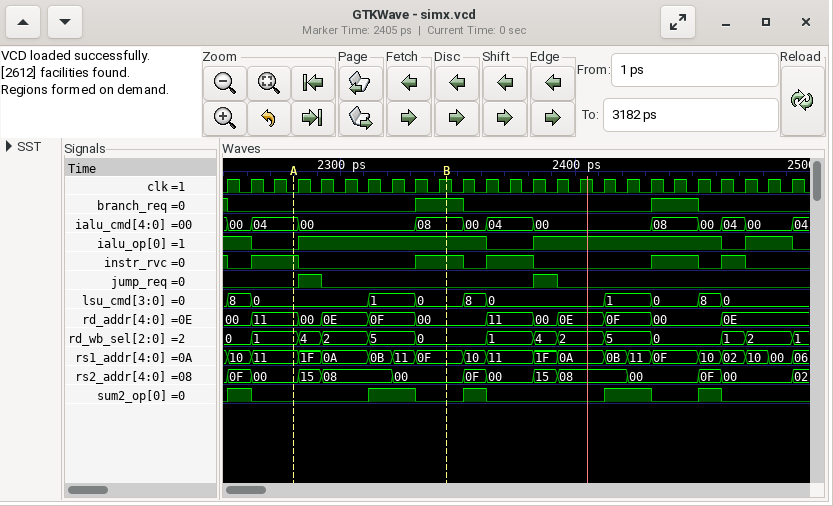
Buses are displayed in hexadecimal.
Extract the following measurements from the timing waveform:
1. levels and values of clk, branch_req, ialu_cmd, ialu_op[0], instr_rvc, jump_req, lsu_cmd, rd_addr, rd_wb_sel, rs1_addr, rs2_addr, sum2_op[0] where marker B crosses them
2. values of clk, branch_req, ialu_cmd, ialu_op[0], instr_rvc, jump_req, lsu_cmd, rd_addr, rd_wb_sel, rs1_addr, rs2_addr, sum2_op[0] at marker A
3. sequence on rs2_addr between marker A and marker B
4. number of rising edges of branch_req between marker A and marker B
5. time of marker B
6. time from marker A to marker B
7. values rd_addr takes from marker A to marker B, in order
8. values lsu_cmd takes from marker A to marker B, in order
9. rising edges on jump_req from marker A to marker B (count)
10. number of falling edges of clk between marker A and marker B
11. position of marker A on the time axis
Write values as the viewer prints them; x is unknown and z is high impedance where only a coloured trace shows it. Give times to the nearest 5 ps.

clk=1, branch_req=1, ialu_cmd=08, ialu_op[0]=1, instr_rvc=1, jump_req=0, lsu_cmd=0, rd_addr=00, rd_wb_sel=0, rs1_addr=0F, rs2_addr=00, sum2_op[0]=0
clk=0, branch_req=0, ialu_cmd=04, ialu_op[0]=0, instr_rvc=1, jump_req=0, lsu_cmd=0, rd_addr=11, rd_wb_sel=1, rs1_addr=11, rs2_addr=00, sum2_op[0]=0
00, 15, 08, 00
1
2345 ps
65 ps
11, 00, 0E, 0F, 00
0, 1, 0
1
6
2280 ps
